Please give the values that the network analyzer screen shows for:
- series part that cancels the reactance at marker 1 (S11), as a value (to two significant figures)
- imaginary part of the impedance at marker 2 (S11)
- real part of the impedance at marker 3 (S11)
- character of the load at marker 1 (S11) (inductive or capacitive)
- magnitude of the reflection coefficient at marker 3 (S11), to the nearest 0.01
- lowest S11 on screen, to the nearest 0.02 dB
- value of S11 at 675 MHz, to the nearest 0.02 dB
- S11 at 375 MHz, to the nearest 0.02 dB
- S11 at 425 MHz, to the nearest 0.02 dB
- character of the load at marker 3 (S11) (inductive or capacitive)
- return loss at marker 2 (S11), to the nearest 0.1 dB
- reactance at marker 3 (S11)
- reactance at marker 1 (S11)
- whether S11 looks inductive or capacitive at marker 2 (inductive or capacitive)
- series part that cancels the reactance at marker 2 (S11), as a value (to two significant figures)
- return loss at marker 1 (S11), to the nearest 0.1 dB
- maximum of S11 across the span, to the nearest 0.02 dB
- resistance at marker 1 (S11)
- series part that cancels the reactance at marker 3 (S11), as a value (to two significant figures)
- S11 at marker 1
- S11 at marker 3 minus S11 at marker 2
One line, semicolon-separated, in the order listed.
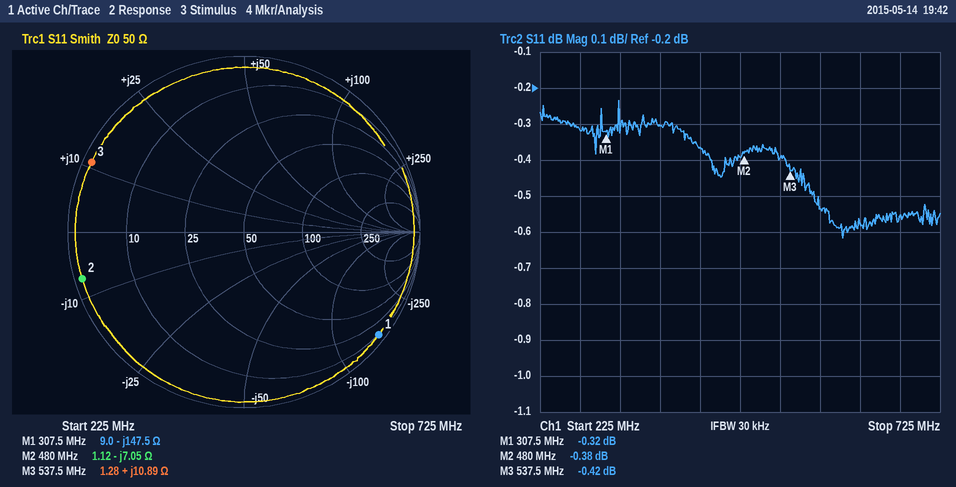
76 nH; -7.05 Ω; 1.28 Ω; capacitive; 0.95; -0.62 dB; -0.56 dB; -0.30 dB; -0.36 dB; inductive; 0.4 dB; +10.89 Ω; -147.5 Ω; capacitive; 2.3 nH; 0.3 dB; -0.24 dB; 9.0 Ω; 27 pF; -0.32 dB; -0.04 dB
